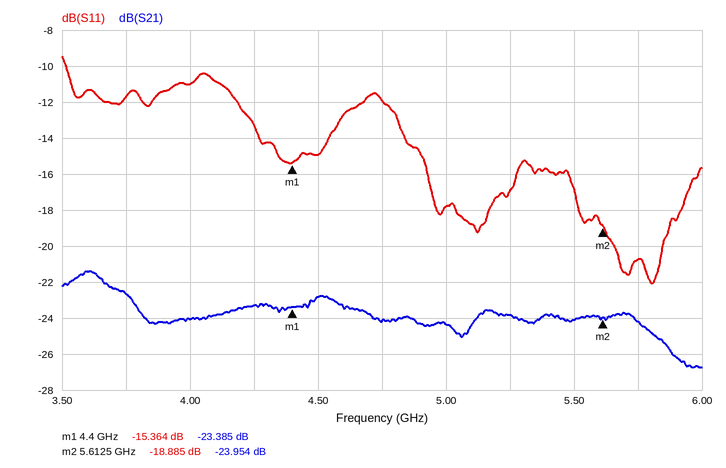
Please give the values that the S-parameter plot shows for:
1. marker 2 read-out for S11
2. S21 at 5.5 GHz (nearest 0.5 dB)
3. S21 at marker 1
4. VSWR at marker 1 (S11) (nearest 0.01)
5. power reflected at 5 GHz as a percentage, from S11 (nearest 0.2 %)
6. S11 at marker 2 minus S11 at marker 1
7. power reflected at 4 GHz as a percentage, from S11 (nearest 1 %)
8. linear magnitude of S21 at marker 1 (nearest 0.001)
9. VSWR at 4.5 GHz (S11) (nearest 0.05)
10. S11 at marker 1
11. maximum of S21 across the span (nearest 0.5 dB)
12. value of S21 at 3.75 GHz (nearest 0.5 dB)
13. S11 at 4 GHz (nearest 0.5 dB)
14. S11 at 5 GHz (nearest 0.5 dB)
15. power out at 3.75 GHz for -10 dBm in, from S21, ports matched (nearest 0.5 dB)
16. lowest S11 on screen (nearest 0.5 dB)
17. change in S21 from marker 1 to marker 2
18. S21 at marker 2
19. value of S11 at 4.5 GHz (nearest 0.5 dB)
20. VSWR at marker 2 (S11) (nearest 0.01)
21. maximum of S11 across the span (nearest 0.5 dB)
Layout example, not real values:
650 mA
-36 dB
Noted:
-18.885 dB
-24.0 dB
-23.385 dB
1.41
1.6 %
-3.521 dB
8 %
0.068
1.45
-15.364 dB
-21.5 dB
-22.5 dB
-11.0 dB
-18.0 dB
-32.5 dBm
-22.0 dB
-0.569 dB
-23.954 dB
-15.0 dB
1.26
-9.5 dB
